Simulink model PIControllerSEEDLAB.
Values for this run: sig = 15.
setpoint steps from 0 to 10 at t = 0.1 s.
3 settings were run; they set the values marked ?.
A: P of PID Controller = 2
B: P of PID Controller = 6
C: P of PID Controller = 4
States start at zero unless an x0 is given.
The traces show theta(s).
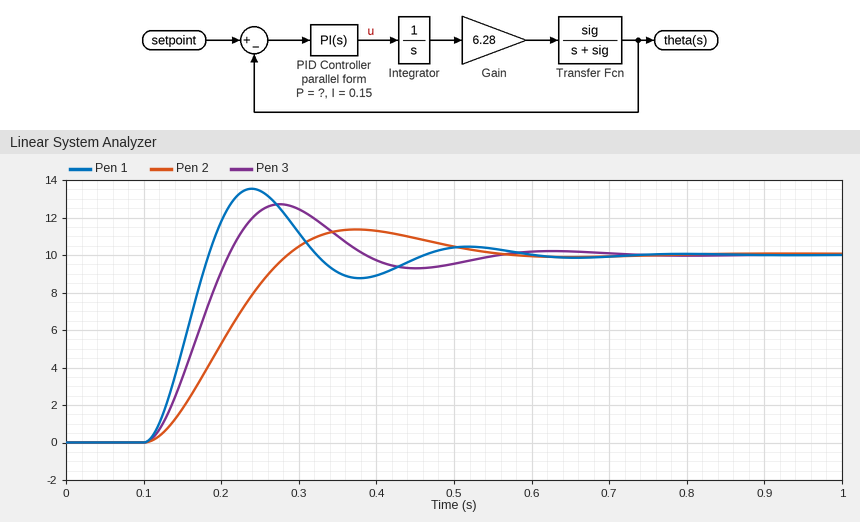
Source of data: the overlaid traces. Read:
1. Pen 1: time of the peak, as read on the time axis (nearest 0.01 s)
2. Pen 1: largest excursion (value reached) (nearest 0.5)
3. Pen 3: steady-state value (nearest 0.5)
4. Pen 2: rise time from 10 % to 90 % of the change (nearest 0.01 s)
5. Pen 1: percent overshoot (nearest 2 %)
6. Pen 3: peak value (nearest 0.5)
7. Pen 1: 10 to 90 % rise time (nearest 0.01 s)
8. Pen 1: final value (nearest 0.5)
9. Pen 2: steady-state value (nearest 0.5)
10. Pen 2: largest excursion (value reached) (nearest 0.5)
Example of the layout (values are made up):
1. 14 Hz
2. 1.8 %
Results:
1. 0.24 s
2. 13.5
3. 10.0
4. 0.13 s
5. 36 %
6. 12.5
7. 0.06 s
8. 10.0
9. 10.0
10. 11.5
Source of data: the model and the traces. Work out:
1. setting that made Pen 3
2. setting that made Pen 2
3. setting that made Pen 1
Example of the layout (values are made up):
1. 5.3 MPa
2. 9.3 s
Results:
1. C
2. A
3. B
